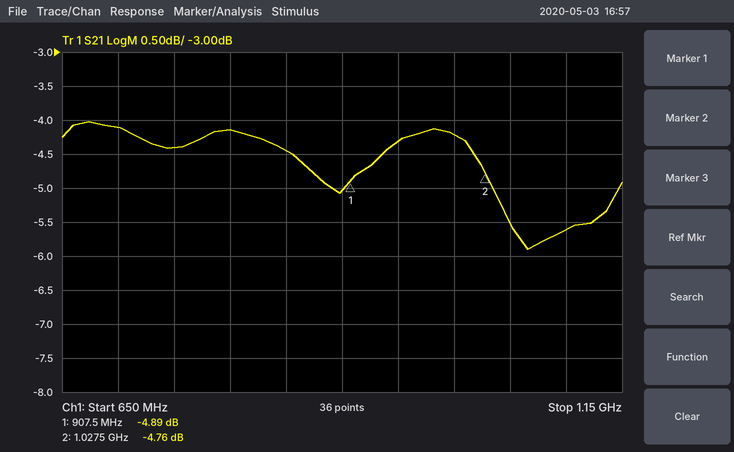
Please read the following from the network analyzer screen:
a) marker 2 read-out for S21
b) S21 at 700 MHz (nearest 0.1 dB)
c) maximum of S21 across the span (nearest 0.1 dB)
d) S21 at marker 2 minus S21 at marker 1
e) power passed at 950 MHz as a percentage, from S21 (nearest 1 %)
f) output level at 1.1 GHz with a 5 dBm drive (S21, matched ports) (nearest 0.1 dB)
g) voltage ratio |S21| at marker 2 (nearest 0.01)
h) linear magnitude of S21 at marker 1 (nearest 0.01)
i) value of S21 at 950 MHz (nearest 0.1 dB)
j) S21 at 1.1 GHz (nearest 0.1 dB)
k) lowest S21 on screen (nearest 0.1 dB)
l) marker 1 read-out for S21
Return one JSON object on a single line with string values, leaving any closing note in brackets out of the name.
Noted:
{"marker 2 read-out for S21": "-4.76 dB", "S21 at 700 MHz": "-4.1 dB", "maximum of S21 across the span": "-4.0 dB", "S21 at marker 2 minus S21 at marker 1": "0.13 dB", "power passed at 950 MHz as a percentage, from S21": "37 %", "output level at 1.1 GHz with a 5 dBm drive (S21, matched ports)": "-0.6 dBm", "voltage ratio |S21| at marker 2": "0.58", "linear magnitude of S21 at marker 1": "0.57", "value of S21 at 950 MHz": "-4.3 dB", "S21 at 1.1 GHz": "-5.6 dB", "lowest S21 on screen": "-5.9 dB", "marker 1 read-out for S21": "-4.89 dB"}
